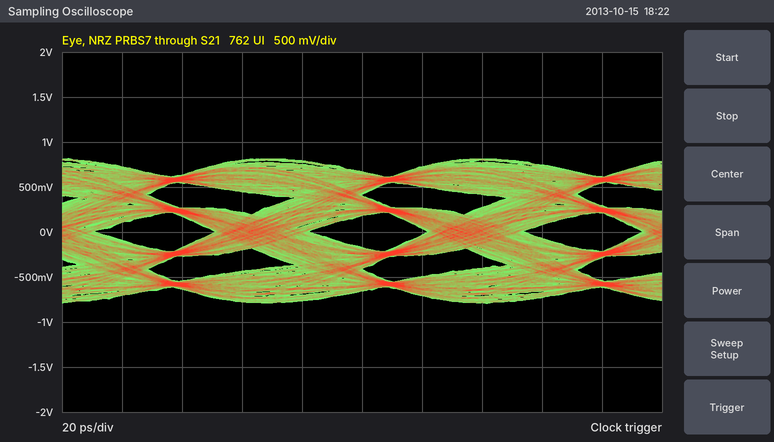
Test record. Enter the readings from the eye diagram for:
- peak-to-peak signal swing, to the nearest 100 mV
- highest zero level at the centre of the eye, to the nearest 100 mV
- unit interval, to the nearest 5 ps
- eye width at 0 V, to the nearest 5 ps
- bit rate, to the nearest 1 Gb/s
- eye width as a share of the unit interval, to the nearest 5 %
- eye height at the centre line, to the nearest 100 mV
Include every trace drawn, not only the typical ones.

1.6 V
-200 mV
70 ps
40 ps
14 Gb/s
55 %
400 mV
